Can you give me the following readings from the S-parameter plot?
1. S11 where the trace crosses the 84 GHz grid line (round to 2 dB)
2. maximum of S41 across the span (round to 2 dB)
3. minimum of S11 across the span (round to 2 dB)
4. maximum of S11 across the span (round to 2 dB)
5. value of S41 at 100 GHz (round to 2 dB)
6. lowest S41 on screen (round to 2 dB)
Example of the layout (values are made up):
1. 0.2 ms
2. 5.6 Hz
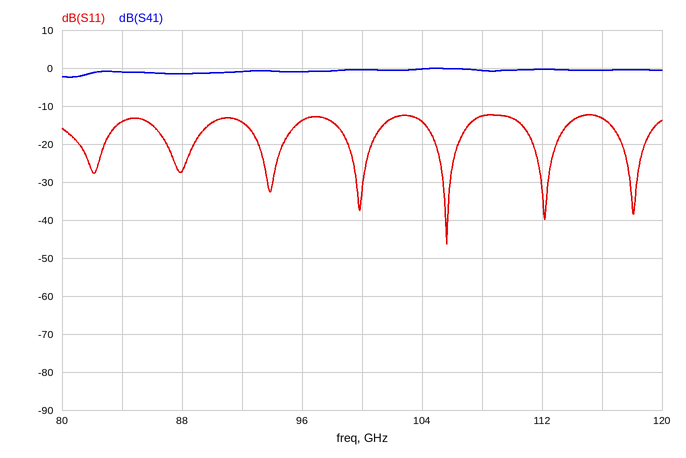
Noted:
1. -14 dB
2. 0 dB
3. -46 dB
4. -12 dB
5. 0 dB
6. -2 dB
